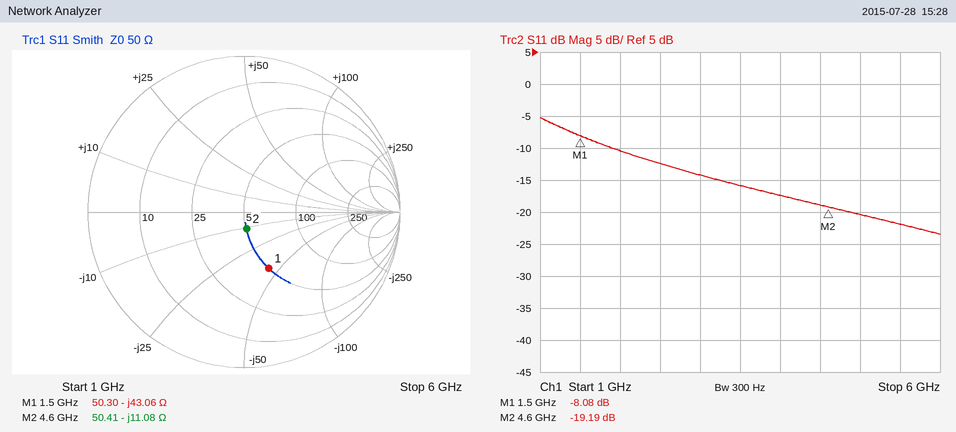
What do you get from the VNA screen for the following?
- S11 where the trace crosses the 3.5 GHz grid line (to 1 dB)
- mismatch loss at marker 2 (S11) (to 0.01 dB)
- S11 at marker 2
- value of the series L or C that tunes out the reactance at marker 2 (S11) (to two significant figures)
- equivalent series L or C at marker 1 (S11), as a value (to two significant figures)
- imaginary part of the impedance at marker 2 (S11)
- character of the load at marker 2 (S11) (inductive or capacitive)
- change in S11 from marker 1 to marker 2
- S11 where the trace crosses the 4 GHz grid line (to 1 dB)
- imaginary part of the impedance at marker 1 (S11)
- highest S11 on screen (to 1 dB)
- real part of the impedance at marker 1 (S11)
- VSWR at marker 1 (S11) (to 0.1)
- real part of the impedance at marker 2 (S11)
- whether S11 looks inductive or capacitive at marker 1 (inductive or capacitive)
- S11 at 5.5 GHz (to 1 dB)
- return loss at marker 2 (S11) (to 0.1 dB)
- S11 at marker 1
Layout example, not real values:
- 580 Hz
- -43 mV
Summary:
- -16 dB
- 0.05 dB
- -19.19 dB
- 380 pH
- 2.5 pF
- -11.08 Ω
- capacitive
- -11.11 dB
- -17 dB
- -43.06 Ω
- -5 dB
- 50.30 Ω
- 2.3
- 50.41 Ω
- capacitive
- -22 dB
- 19.2 dB
- -8.08 dB
